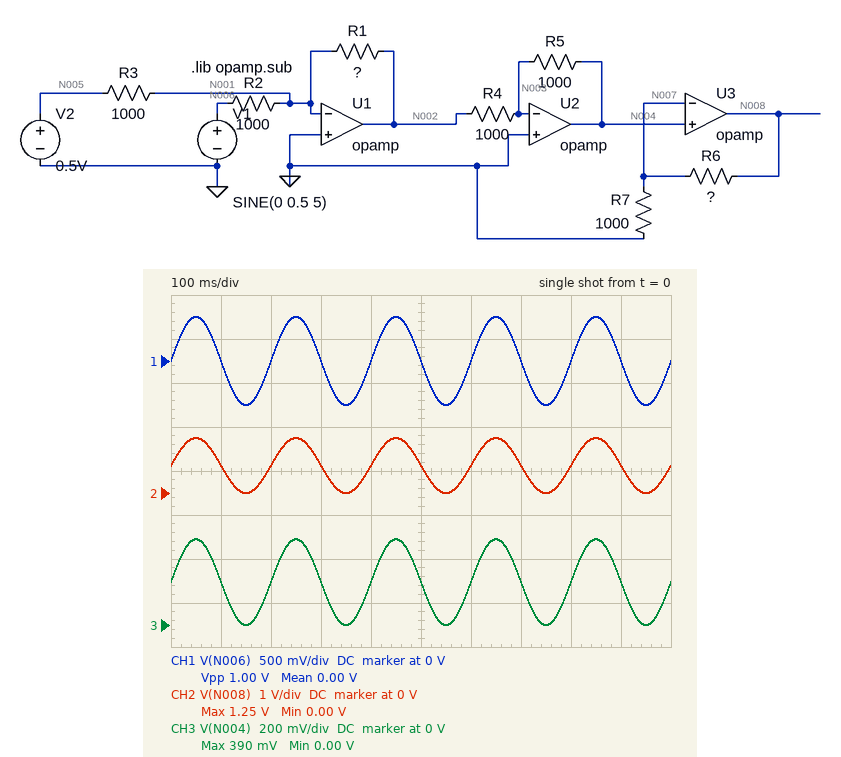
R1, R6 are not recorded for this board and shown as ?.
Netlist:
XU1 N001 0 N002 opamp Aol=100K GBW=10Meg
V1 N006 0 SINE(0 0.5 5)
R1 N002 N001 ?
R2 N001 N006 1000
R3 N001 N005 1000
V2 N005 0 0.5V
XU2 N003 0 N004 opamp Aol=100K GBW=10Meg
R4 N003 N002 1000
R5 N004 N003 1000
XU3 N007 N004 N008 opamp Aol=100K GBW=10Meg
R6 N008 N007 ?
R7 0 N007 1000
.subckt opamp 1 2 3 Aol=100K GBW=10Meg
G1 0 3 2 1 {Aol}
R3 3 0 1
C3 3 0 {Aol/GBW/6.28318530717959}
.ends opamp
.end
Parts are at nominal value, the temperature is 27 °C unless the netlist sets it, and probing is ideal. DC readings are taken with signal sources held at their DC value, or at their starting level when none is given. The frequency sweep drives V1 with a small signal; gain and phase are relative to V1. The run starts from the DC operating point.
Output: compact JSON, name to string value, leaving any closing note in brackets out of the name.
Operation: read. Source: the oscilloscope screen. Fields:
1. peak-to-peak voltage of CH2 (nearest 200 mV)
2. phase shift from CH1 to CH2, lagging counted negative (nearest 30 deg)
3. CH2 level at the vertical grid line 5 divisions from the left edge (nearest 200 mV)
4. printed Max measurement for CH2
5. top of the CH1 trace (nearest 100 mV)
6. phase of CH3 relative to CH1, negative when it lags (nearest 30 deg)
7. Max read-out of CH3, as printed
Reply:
{"peak-to-peak voltage of CH2": "1.2 V", "phase shift from CH1 to CH2, lagging counted negative": "0 deg", "CH2 level at the vertical grid line 5 divisions from the left edge": "600 mV", "printed Max measurement for CH2": "1.25 V", "top of the CH1 trace": "500 mV", "phase of CH3 relative to CH1, negative when it lags": "0 deg", "Max read-out of CH3, as printed": "390 mV"}
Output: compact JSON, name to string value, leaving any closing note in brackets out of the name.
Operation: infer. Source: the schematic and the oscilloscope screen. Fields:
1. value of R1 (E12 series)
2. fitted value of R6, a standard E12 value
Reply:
{"value of R1": "390 Ω", "fitted value of R6, a standard E12 value": "2.2 kΩ"}
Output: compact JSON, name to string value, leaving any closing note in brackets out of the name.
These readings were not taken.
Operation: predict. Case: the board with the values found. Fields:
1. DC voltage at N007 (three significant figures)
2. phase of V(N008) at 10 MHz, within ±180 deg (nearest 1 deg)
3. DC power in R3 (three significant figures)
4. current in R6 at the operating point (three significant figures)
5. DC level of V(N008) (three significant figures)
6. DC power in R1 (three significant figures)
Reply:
{"DC voltage at N007": "195 mV", "phase of V(N008) at 10 MHz, within ±180 deg": "163 deg", "DC power in R3": "250 µW", "current in R6 at the operating point": "195 µA", "DC level of V(N008)": "624 mV", "DC power in R1": "97.5 µW"}
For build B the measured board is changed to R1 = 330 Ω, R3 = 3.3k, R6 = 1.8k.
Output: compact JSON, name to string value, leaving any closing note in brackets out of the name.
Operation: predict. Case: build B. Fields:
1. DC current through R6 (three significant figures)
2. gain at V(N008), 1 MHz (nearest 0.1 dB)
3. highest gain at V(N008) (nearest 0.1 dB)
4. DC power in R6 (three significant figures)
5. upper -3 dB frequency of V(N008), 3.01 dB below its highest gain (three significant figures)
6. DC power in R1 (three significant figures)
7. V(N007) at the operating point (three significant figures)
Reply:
{"DC current through R6": "50.0 µA", "gain at V(N008), 1 MHz": "-1.3 dB", "highest gain at V(N008)": "-0.7 dB", "DC power in R6": "4.50 µW", "upper -3 dB frequency of V(N008), 3.01 dB below its highest gain": "2.40 MHz", "DC power in R1": "7.58 µW", "V(N007) at the operating point": "50.0 mV"}
